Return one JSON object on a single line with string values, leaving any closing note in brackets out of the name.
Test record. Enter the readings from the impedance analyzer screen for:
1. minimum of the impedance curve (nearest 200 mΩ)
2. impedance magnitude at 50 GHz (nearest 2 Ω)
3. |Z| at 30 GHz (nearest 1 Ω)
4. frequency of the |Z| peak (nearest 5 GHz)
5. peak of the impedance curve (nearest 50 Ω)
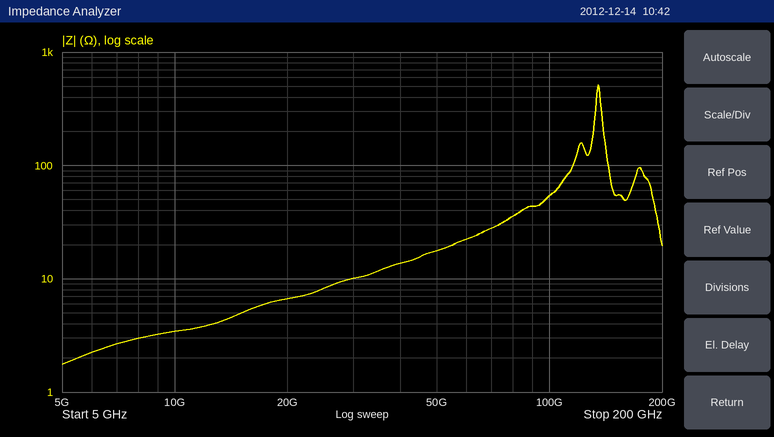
{"minimum of the impedance curve": "1.8 Ω", "impedance magnitude at 50 GHz": "18 Ω", "|Z| at 30 GHz": "10 Ω", "frequency of the |Z| peak": "135 GHz", "peak of the impedance curve": "500 Ω"}
